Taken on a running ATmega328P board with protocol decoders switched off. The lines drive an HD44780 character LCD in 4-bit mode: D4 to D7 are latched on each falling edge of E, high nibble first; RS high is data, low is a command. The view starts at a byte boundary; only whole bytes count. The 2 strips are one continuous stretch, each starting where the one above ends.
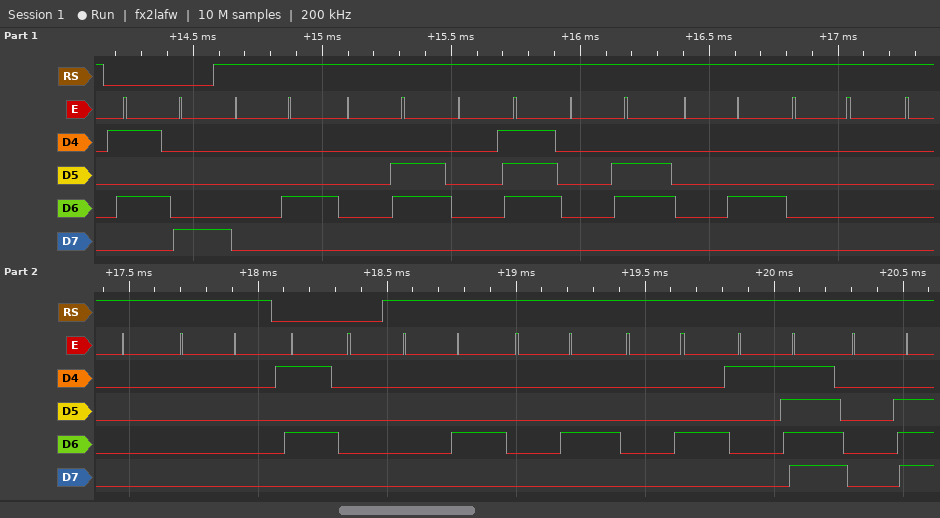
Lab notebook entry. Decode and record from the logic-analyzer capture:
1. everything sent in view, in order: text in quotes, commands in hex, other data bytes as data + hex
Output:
0x58 data 04 06 07 06 04 00 00 00 0x50 data 04 04 04 1F 0E
